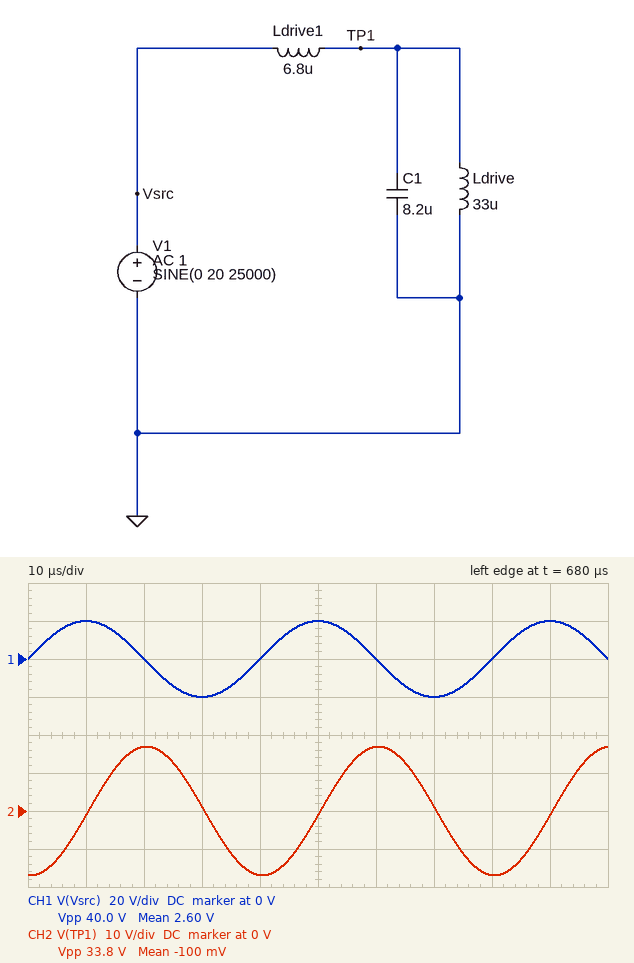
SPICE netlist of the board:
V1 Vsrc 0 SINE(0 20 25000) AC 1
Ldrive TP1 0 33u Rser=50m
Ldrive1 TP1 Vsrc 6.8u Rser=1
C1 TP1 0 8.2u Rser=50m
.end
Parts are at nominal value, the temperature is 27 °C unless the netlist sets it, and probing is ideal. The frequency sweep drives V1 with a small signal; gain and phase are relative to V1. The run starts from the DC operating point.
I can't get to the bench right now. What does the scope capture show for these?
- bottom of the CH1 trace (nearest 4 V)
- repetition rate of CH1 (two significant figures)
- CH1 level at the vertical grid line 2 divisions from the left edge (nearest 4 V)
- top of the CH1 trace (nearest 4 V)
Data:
-20 V
25 kHz
0 V
20 V
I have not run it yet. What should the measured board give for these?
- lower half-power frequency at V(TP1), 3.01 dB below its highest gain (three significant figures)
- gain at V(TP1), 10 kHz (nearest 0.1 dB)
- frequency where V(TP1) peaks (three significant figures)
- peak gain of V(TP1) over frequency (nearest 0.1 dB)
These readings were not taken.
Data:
6.26 kHz
-0.1 dB
16.7 kHz
1.2 dB
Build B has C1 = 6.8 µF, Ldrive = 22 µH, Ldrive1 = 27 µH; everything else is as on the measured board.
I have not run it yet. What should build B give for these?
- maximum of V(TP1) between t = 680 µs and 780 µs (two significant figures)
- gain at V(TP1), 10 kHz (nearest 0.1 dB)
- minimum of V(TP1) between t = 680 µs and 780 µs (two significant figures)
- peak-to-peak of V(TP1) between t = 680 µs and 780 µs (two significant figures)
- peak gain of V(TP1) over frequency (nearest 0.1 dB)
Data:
8.1 V
-3.8 dB
-8.1 V
16 V
7.2 dB
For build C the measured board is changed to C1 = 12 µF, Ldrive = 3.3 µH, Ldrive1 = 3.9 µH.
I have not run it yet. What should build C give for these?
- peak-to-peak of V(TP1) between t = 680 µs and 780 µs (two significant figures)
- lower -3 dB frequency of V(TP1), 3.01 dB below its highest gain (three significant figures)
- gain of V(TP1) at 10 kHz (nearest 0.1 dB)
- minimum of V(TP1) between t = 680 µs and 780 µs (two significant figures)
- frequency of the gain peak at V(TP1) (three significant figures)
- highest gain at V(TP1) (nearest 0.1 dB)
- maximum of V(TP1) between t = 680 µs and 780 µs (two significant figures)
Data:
29 V
21.1 kHz
-13.4 dB
-14 V
28.5 kHz
-2.1 dB
14 V
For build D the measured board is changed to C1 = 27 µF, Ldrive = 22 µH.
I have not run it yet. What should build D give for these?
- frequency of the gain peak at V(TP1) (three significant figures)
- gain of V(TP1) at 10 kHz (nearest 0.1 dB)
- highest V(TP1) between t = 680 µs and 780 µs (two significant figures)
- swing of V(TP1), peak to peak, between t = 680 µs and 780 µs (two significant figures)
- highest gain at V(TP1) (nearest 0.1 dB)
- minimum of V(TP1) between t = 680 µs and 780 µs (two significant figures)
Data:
7.46 kHz
-2.2 dB
3.9 V
7.7 V
-0.7 dB
-3.9 V
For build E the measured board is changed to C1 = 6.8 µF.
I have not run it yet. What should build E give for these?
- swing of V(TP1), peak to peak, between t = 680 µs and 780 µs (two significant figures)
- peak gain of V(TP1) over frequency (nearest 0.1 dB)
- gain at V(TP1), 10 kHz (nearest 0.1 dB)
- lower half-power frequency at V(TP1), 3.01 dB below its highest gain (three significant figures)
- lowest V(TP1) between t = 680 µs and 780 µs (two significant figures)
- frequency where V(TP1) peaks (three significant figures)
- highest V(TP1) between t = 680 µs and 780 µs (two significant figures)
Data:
42 V
1.7 dB
-0.4 dB
7.55 kHz
-21 V
19.6 kHz
21 V
